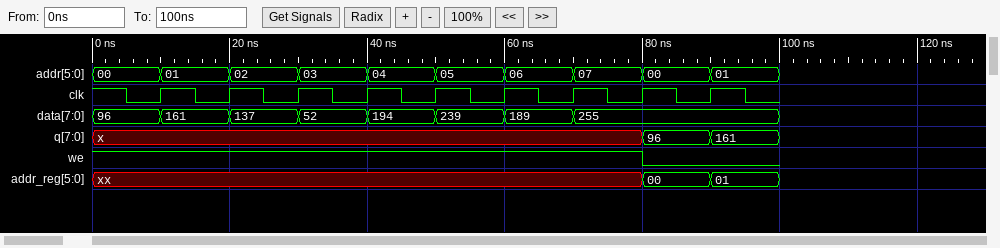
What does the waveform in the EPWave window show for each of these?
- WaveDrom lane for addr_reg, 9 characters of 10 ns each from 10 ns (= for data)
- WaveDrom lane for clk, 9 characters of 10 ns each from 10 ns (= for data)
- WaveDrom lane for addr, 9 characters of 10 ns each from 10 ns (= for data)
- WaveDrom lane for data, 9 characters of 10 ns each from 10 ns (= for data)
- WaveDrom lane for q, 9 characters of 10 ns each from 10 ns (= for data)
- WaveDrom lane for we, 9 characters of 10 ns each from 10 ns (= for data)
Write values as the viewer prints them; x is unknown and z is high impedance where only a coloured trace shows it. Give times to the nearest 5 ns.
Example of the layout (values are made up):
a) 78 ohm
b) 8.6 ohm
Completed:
a) {name: 'addr_reg', wave: 'x......==', data: '00 01'}
b) {name: 'clk', wave: 'p........'}
c) {name: 'addr', wave: '=========', data: '01 02 03 04 05 06 07 00 01'}
d) {name: 'data', wave: '=======..', data: '161 137 52 194 239 189 255'}
e) {name: 'q', wave: 'x......==', data: '96 161'}
f) {name: 'we', wave: '1......0.'}
